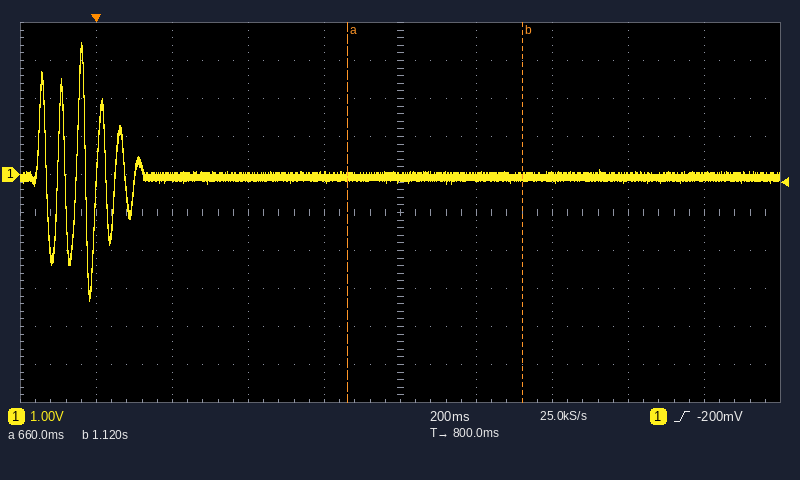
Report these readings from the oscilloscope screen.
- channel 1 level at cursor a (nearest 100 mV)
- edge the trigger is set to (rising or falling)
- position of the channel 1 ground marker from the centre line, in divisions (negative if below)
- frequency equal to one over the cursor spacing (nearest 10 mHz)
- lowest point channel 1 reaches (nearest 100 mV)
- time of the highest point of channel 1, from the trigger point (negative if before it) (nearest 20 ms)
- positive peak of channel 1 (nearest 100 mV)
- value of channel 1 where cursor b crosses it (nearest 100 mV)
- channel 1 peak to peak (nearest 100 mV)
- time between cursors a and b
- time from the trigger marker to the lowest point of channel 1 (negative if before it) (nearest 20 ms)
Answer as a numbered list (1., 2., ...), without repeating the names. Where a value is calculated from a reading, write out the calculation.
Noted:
1. -100 mV
2. rising
3. +1.0 div
4. 1 / 460 ms ≈ 2.17 Hz
5. -3.3 V
6. -40 ms
7. 3.5 V
8. -100 mV
9. 3.5 V − (-3.3 V) = 6.8 V
10. 1.12 s − (660 ms) = 460 ms
11. -20 ms
